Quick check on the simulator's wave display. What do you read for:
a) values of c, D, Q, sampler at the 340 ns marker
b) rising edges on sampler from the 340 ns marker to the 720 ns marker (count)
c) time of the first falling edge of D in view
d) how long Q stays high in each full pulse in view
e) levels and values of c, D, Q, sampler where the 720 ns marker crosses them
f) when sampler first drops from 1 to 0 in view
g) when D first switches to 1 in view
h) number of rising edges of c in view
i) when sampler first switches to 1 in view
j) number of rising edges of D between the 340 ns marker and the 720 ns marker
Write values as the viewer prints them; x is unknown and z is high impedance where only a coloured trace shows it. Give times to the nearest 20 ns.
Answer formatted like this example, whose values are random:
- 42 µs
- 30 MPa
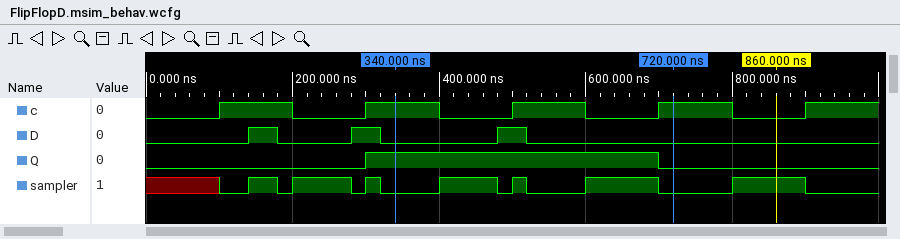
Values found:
- c=1, D=0, Q=1, sampler=0
- 3
- 180 ns
- 400 ns
- c=1, D=0, Q=0, sampler=0
- 180 ns
- 140 ns
- 5
- 140 ns
- 1
